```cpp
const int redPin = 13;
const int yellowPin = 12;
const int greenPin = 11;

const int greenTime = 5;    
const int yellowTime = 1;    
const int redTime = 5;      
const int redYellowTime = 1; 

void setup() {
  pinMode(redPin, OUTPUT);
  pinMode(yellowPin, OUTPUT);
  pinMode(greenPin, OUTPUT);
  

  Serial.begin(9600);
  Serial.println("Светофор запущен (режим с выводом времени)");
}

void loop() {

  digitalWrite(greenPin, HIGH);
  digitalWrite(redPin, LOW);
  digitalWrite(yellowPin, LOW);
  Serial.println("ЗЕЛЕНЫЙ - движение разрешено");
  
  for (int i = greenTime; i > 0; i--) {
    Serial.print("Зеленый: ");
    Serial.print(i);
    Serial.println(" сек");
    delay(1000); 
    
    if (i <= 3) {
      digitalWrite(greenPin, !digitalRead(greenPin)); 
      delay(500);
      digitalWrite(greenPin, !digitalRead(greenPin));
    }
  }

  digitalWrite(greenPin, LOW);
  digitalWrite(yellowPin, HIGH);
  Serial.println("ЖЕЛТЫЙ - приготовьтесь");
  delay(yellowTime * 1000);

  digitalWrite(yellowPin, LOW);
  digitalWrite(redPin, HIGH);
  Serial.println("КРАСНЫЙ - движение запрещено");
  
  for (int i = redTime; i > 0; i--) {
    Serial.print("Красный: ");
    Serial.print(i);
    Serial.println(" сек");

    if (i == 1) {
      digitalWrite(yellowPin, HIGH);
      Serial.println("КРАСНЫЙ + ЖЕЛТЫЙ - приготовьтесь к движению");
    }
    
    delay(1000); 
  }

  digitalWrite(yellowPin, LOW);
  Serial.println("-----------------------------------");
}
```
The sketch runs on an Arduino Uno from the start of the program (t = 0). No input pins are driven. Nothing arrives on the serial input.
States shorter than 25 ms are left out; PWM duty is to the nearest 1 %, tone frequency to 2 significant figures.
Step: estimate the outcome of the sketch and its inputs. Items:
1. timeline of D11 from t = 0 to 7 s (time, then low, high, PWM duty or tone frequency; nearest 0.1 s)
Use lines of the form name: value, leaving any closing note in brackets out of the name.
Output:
timeline of D11 from t = 0 to 7 s: 0 s high; 3.1 s low; 3.6 s high; 4.6 s low; 5.1 s high; 6.1 s low
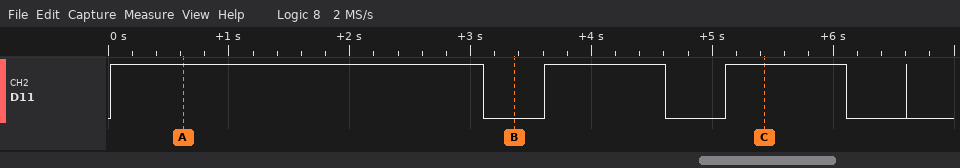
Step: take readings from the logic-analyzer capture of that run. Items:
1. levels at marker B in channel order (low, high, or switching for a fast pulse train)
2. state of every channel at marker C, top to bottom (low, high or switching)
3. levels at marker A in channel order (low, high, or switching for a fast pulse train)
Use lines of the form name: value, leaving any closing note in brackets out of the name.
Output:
levels at marker B in channel order: D11 low
state of every channel at marker C, top to bottom: D11 high
levels at marker A in channel order: D11 high
